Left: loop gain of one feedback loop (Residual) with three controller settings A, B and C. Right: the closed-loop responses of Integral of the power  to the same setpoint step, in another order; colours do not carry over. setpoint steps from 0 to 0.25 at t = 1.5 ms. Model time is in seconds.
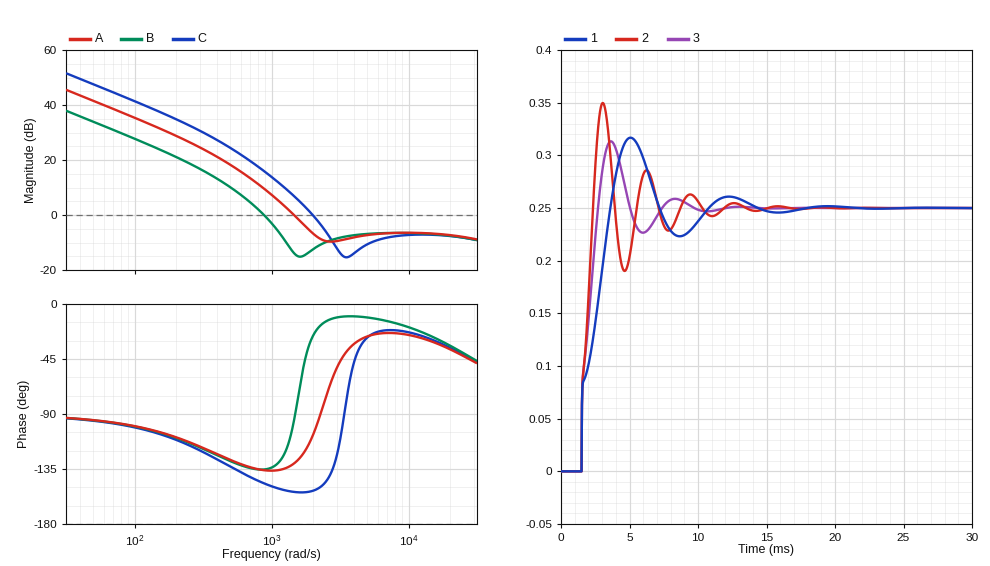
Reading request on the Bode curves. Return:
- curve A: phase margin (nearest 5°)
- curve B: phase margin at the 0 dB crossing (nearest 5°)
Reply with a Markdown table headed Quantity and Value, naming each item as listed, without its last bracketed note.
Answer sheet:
| Quantity | Value |
|---|---|
| curve A: phase margin | 50° |
| curve B: phase margin at the 0 dB crossing | 45° |
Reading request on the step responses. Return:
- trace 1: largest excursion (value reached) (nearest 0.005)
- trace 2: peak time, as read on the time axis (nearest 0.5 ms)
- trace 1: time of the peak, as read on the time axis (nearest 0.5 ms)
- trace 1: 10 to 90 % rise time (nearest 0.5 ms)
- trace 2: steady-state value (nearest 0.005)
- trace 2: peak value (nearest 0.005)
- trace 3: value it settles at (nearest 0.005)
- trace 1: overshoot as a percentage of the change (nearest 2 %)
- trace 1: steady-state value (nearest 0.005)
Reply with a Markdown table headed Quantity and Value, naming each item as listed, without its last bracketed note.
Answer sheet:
| Quantity | Value |
|---|---|
| trace 1: largest excursion (value reached) | 0.315 |
| trace 2: peak time, as read on the time axis | 3.0 ms |
| trace 1: time of the peak, as read on the time axis | 5.0 ms |
| trace 1: 10 to 90 % rise time | 2.0 ms |
| trace 2: steady-state value | 0.250 |
| trace 2: peak value | 0.350 |
| trace 3: value it settles at | 0.250 |
| trace 1: overshoot as a percentage of the change | 26 % |
| trace 1: steady-state value | 0.250 |
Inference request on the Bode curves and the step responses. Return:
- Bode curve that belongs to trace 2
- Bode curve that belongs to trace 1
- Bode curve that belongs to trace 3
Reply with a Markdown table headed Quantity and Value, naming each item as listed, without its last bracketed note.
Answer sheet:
| Quantity | Value |
|---|---|
| Bode curve that belongs to trace 2 | C |
| Bode curve that belongs to trace 1 | B |
| Bode curve that belongs to trace 3 | A |
